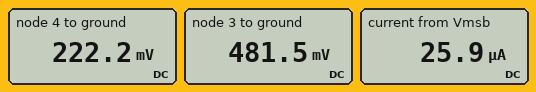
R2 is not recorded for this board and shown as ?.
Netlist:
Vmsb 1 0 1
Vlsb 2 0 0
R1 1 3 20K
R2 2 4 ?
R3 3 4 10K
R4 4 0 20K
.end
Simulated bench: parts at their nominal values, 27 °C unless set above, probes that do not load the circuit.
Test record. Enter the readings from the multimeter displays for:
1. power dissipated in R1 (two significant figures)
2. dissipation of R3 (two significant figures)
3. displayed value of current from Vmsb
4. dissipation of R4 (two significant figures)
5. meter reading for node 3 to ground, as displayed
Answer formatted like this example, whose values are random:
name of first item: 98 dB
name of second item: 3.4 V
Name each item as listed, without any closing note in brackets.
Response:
power dissipated in R1: 13 µW
dissipation of R3: 6.7 µW
displayed value of current from Vmsb: 25.9 µA
dissipation of R4: 2.5 µW
meter reading for node 3 to ground, as displayed: 481.5 mV
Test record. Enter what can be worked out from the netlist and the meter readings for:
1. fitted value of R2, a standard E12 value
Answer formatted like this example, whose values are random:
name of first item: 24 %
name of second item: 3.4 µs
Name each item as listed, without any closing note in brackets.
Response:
fitted value of R2, a standard E12 value: 15 kΩ
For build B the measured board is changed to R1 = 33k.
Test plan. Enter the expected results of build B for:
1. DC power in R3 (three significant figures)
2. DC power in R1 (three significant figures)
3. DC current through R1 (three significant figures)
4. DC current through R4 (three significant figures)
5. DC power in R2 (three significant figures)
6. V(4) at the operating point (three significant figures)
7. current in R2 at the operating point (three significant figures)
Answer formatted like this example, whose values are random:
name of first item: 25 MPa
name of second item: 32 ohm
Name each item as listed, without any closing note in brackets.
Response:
DC power in R3: 3.76 µW
DC power in R1: 12.4 µW
DC current through R1: 19.4 µA
DC current through R4: 8.31 µA
DC power in R2: 1.84 µW
V(4) at the operating point: 166 mV
current in R2 at the operating point: 11.1 µA
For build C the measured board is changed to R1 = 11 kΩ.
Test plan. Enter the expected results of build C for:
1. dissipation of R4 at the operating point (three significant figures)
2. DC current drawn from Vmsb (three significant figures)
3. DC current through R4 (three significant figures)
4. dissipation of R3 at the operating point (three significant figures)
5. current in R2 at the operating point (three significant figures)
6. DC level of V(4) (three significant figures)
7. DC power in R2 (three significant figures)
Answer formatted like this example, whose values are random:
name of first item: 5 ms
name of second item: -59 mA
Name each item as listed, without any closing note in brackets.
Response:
dissipation of R4 at the operating point: 4.20 µW
DC current drawn from Vmsb: 33.8 µA
DC current through R4: 14.5 µA
dissipation of R3 at the operating point: 11.4 µW
current in R2 at the operating point: 19.3 µA
DC level of V(4): 290 mV
DC power in R2: 5.60 µW
